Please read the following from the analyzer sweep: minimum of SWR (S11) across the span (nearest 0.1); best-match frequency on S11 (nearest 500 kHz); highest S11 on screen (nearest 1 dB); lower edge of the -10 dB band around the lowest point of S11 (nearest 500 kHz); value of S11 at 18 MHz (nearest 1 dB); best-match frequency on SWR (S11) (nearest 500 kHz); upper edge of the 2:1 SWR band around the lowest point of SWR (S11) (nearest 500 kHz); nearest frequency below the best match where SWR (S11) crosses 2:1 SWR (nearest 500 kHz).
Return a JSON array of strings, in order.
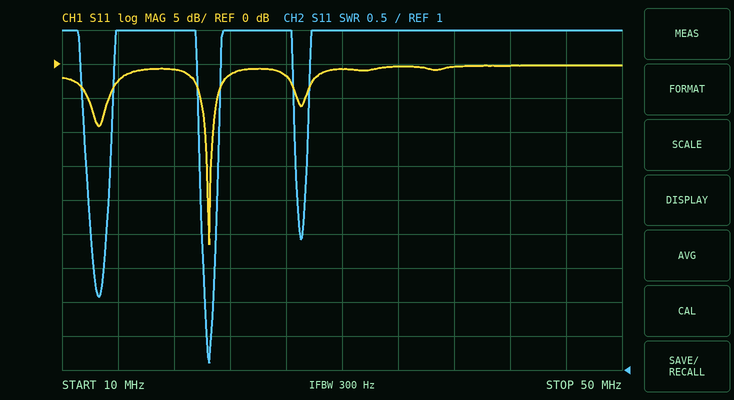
["1.1", "20.5 MHz", "0 dB", "20.0 MHz", "-1 dB", "20.5 MHz", "21.0 MHz", "20.0 MHz"]
